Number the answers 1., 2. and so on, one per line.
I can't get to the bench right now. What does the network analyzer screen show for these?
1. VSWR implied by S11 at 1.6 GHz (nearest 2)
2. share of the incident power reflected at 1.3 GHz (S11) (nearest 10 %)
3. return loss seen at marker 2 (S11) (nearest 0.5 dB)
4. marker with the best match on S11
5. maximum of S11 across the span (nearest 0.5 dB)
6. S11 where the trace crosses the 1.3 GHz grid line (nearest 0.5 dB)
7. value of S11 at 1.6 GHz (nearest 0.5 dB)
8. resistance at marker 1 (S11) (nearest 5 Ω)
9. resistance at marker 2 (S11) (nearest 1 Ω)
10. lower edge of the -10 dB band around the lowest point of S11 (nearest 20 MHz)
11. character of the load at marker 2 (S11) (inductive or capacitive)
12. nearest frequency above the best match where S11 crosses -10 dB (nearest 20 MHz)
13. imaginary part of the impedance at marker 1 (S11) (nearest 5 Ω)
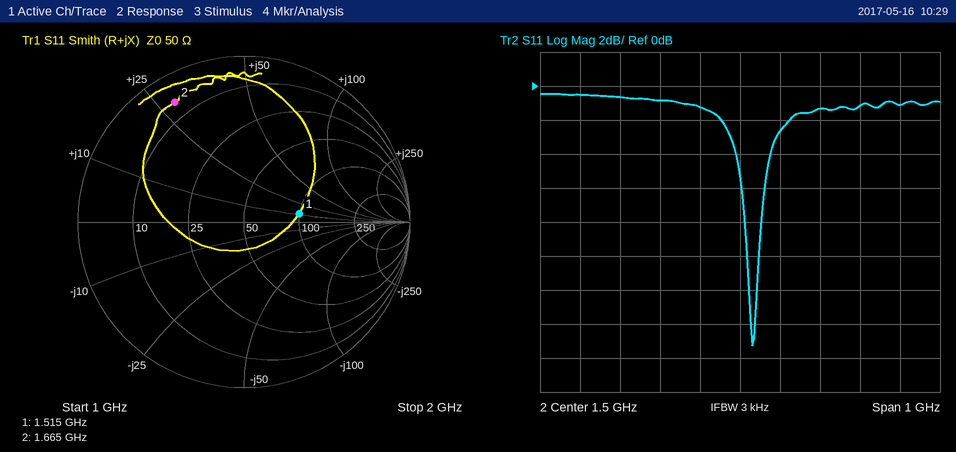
1. 6
2. 80 %
3. 1.5 dB
4. marker 1
5. -0.5 dB
6. -1.0 dB
7. -2.5 dB
8. 100 Ω
9. 6 Ω
10. 1.52 GHz
11. inductive
12. 1.54 GHz
13. +10 Ω
